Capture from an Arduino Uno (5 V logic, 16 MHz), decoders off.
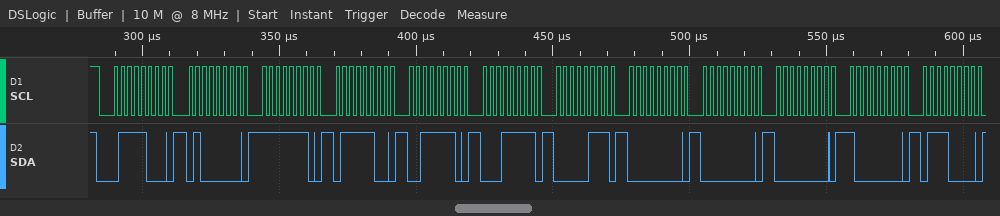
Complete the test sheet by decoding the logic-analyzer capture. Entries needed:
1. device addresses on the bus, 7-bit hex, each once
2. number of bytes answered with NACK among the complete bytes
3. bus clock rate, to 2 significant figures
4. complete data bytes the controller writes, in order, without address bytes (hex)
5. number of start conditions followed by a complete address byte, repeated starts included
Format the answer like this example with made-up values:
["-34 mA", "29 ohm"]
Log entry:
["0x3C", "0", "400 kHz", "40 FE 7C 3E 1F 07 00 00 00 80 70", "1"]
